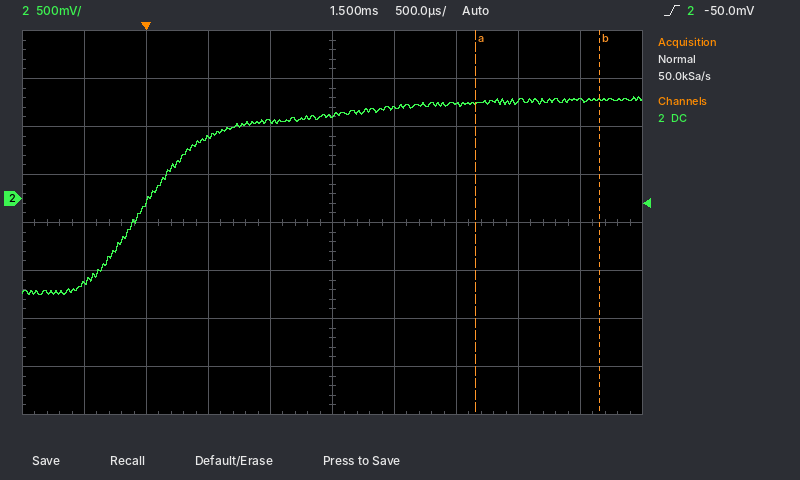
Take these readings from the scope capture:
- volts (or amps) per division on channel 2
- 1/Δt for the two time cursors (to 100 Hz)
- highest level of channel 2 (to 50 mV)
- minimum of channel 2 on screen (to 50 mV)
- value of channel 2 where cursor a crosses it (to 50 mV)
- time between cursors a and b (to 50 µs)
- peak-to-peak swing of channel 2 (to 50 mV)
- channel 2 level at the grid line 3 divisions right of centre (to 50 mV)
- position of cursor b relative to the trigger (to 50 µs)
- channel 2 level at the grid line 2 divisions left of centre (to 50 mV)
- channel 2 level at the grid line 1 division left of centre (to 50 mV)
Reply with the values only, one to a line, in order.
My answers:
500 mV
1.0 kHz
1.05 V
-1.00 V
1.00 V
1.00 ms
2.05 V
1.00 V
+3.65 ms
650 mV
800 mV
